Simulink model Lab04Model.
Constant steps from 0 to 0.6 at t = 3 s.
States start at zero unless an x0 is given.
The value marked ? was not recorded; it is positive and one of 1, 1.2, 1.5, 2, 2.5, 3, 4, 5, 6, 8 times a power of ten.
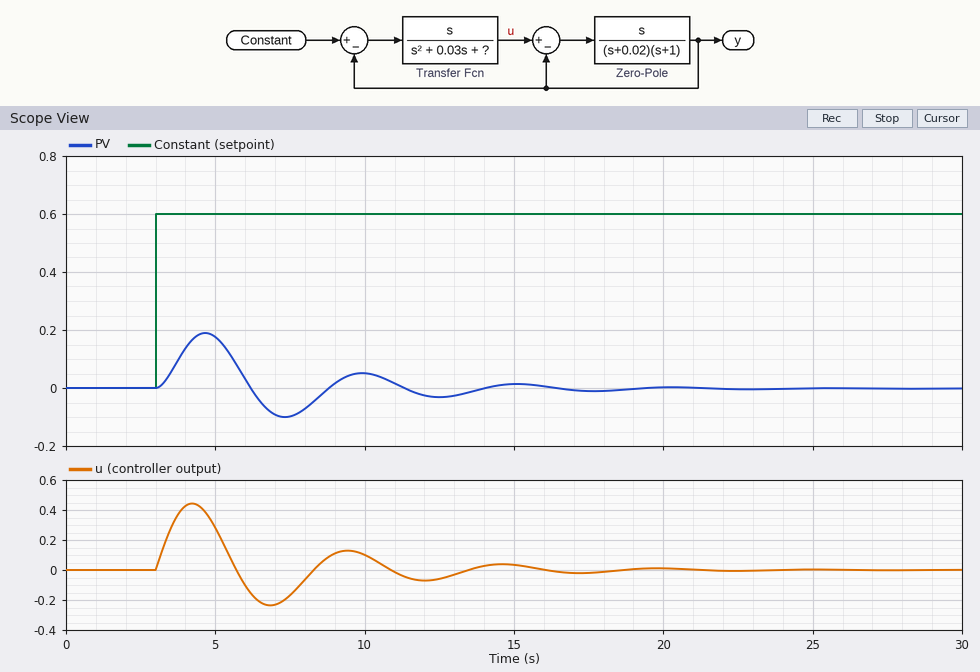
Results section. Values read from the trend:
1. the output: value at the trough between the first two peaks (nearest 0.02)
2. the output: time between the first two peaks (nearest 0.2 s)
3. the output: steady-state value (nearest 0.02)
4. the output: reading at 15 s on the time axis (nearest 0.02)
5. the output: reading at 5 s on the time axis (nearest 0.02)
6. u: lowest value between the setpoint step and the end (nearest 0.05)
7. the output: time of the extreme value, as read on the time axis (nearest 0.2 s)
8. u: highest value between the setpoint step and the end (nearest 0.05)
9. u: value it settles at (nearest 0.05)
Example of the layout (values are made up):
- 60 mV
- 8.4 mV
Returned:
- -0.10
- 5.2 s
- 0.00
- 0.02
- 0.18
- -0.25
- 4.6 s
- 0.45
- 0.00
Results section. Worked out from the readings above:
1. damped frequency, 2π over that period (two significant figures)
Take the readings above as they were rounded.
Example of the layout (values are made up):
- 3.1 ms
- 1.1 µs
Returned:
- 1.2 rad/s
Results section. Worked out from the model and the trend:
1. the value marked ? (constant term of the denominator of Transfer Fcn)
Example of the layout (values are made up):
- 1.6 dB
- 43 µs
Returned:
- 1.2
